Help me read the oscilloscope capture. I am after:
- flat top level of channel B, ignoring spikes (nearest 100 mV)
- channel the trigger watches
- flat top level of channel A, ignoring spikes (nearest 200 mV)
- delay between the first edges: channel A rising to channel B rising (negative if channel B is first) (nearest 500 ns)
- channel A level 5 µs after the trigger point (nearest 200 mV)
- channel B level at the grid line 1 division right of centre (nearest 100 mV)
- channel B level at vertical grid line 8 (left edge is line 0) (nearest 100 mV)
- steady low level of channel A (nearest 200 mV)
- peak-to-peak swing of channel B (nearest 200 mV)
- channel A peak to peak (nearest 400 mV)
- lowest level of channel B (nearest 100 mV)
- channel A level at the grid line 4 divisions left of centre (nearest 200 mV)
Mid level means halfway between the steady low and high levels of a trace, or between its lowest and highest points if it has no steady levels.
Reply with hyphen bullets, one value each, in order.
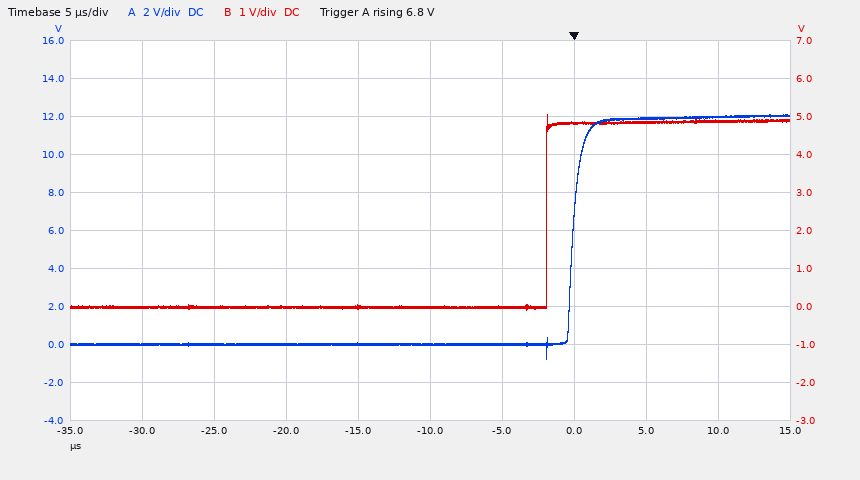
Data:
- 4.9 V
- channel A
- 12.0 V
- -2.0 µs
- 12.0 V
- 0.0 V
- 4.9 V
- 0.0 V
- 5.2 V
- 12.8 V
- -100 mV
- 0.0 V
